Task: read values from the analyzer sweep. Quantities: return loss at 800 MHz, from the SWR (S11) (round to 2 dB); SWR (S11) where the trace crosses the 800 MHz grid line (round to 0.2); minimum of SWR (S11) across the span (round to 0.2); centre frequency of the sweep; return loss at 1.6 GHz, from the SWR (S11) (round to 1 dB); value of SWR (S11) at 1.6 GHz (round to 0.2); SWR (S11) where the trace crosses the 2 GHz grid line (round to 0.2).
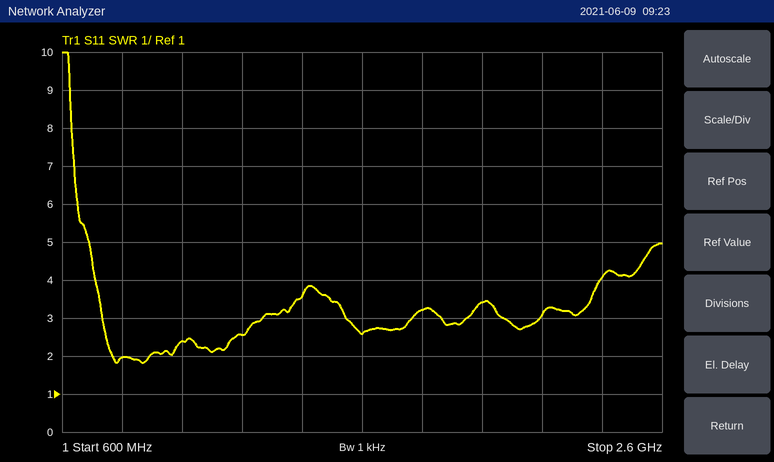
10 dB
2.0
1.8
1.6 GHz
7 dB
2.6
3.4
